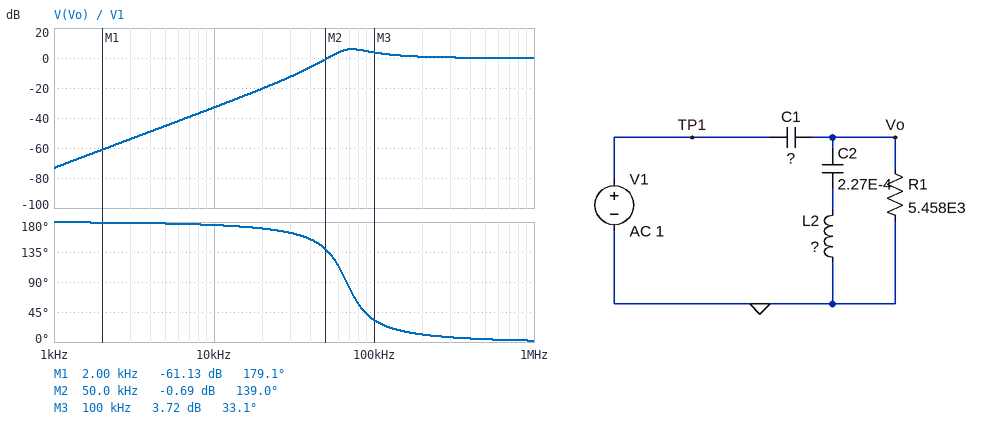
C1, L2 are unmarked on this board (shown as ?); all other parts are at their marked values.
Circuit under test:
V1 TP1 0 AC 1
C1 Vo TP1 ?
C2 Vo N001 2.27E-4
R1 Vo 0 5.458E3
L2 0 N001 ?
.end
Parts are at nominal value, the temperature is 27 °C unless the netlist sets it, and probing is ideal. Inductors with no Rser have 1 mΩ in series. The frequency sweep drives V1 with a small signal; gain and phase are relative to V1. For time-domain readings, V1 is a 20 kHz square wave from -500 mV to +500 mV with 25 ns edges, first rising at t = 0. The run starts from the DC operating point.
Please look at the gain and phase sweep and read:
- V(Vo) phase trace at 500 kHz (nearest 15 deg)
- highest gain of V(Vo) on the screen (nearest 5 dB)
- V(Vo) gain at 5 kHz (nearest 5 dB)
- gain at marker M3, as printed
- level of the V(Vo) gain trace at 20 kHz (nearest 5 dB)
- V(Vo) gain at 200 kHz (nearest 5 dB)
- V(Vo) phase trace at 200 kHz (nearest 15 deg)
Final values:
0 deg
5 dB
-45 dB
3.72 dB
-20 dB
0 dB
15 deg
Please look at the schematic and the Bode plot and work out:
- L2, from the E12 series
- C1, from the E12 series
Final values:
6.8 mH
820 pF
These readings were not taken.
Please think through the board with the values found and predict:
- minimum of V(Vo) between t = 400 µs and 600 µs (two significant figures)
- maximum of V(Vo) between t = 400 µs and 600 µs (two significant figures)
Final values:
-1.0 V
1.0 V
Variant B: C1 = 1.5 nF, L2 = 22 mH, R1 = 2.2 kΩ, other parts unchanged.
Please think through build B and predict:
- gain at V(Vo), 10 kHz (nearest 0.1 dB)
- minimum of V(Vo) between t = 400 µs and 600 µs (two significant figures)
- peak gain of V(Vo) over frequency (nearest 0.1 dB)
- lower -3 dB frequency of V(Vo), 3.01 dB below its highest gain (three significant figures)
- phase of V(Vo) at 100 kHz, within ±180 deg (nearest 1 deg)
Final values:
-18.3 dB
-1.0 V
0 dB
35.5 kHz
28 deg
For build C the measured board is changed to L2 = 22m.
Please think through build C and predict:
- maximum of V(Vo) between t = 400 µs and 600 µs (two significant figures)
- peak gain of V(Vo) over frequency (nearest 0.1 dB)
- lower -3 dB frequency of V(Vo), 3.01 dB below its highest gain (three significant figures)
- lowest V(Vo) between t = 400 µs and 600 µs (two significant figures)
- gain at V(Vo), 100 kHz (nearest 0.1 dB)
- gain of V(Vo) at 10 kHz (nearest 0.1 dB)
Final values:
940 mV
1.6 dB
31.8 kHz
-940 mV
0.6 dB
-22.6 dB
